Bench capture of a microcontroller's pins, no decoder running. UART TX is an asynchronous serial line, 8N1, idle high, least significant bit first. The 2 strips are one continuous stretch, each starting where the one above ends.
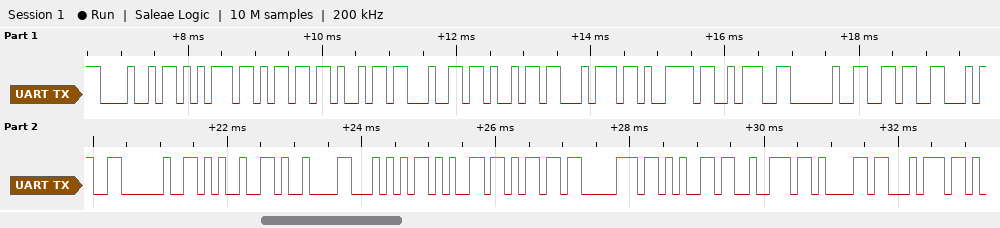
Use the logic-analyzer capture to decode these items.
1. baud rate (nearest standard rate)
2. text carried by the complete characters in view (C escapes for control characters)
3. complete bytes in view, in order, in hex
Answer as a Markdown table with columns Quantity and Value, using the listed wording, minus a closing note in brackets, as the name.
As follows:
| Quantity | Value |
|---|---|
| baud rate | 9600 baud |
| text carried by the complete characters in view | "Humidity: 64 %\tTemperat" |
| complete bytes in view, in order, in hex | 0x48 0x75 0x6D 0x69 0x64 0x69 0x74 0x79 0x3A 0x20 0x36 0x34 0x20 0x25 0x09 0x54 0x65 0x6D 0x70 0x65 0x72 0x61 0x74 |
